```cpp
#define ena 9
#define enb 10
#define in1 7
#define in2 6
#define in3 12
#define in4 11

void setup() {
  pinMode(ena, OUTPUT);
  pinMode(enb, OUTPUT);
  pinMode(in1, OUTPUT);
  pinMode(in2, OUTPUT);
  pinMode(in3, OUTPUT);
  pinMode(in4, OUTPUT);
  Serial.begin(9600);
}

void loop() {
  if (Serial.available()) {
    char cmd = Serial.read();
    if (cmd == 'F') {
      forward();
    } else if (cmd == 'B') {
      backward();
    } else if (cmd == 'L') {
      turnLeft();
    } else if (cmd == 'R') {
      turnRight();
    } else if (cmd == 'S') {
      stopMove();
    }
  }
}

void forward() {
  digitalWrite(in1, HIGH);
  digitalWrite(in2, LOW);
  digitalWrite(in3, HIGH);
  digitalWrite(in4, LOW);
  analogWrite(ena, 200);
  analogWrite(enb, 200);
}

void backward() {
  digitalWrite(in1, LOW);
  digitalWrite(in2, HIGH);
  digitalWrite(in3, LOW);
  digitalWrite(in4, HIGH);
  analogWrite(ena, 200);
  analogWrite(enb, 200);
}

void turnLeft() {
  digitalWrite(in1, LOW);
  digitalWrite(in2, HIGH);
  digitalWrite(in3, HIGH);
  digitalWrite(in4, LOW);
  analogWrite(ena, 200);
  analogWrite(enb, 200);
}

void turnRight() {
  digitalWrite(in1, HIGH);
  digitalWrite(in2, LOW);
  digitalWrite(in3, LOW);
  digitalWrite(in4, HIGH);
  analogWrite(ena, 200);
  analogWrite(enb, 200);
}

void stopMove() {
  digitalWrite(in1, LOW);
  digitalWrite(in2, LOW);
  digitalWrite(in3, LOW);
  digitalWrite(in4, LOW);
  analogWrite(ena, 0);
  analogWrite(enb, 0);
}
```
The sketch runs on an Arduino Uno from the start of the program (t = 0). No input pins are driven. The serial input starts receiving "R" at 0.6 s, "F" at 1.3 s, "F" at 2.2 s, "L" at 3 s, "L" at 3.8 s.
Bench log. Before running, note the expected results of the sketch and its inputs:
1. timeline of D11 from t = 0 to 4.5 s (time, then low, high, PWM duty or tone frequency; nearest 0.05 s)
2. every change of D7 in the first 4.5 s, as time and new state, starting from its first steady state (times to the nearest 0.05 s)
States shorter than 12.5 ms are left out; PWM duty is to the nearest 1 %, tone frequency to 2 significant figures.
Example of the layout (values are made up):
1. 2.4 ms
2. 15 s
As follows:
1. 0 s low; 0.6 s high; 1.3 s low
2. 0 s low; 0.6 s high; 3 s low
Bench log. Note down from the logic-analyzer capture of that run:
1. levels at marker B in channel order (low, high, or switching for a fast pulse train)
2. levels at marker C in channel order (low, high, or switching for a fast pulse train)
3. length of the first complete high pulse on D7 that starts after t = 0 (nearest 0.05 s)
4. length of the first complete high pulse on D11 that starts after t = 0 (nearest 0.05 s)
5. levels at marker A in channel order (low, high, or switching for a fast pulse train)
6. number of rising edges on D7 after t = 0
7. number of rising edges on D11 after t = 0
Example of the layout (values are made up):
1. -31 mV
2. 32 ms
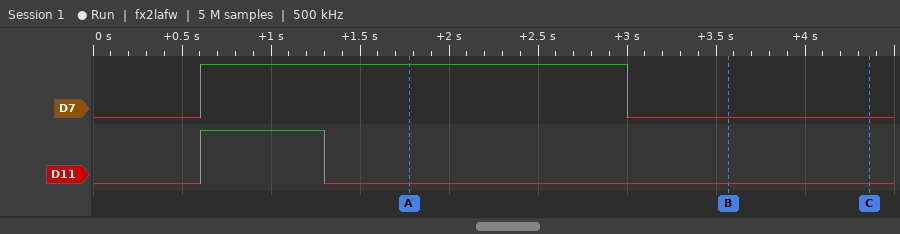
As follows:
1. D7 low, D11 low
2. D7 low, D11 low
3. 2.40 s
4. 0.70 s
5. D7 high, D11 low
6. 1
7. 1
